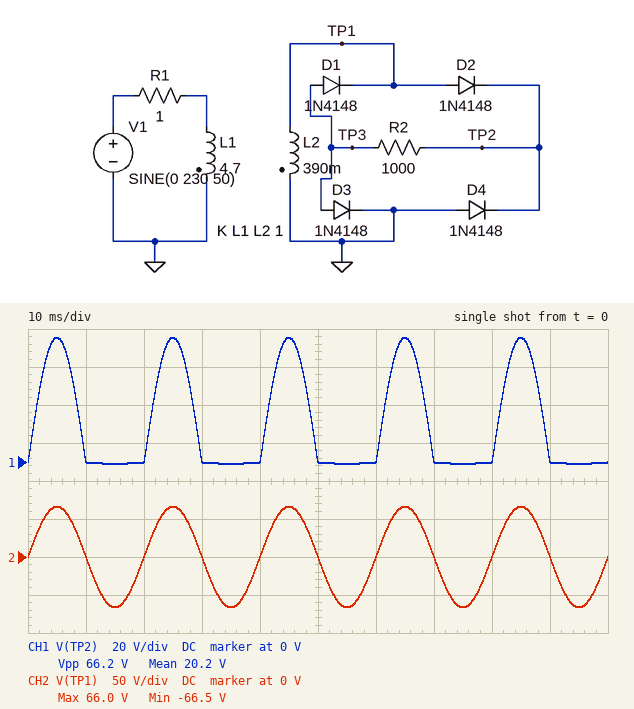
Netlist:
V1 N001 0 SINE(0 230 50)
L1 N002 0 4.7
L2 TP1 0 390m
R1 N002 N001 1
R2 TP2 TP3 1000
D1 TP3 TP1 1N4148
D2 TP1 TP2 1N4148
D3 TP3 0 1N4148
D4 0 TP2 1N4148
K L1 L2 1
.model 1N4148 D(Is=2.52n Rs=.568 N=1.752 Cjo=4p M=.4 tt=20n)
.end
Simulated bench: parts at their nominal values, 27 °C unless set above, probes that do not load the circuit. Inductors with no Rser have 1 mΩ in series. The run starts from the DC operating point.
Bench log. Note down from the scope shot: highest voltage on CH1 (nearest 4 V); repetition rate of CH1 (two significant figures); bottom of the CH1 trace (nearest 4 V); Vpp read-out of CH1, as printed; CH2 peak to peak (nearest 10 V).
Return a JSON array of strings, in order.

["64 V", "50 Hz", "0 V", "66.2 V", "130 V"]
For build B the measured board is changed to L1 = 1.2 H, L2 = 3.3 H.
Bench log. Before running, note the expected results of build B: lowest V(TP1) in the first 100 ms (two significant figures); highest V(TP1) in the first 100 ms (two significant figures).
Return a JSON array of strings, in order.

["-380 V", "380 V"]
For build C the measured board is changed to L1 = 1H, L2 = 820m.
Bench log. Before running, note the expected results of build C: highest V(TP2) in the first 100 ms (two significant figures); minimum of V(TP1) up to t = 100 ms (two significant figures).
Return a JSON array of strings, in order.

["210 V", "-210 V"]
